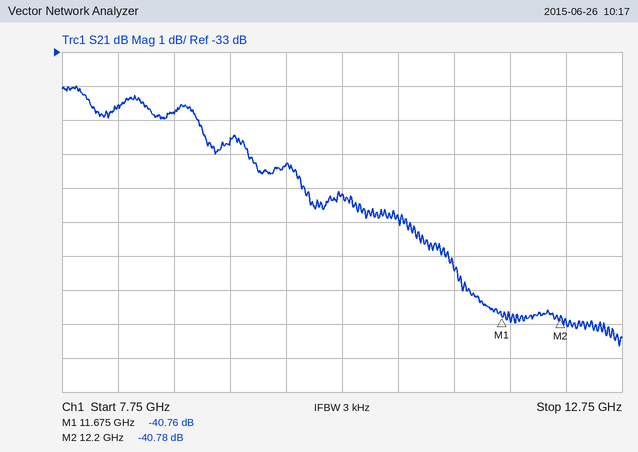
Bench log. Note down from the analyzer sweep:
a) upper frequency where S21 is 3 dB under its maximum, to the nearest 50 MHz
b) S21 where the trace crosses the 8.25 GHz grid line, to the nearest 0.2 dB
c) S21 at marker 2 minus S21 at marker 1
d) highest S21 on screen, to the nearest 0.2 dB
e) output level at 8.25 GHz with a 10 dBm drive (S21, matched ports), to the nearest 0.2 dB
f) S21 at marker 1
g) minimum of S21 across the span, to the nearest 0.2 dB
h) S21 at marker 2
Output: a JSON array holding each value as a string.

["9.90 GHz", "-34.6 dB", "-0.02 dB", "-34.0 dB", "-24.6 dBm", "-40.76 dB", "-41.6 dB", "-40.78 dB"]
